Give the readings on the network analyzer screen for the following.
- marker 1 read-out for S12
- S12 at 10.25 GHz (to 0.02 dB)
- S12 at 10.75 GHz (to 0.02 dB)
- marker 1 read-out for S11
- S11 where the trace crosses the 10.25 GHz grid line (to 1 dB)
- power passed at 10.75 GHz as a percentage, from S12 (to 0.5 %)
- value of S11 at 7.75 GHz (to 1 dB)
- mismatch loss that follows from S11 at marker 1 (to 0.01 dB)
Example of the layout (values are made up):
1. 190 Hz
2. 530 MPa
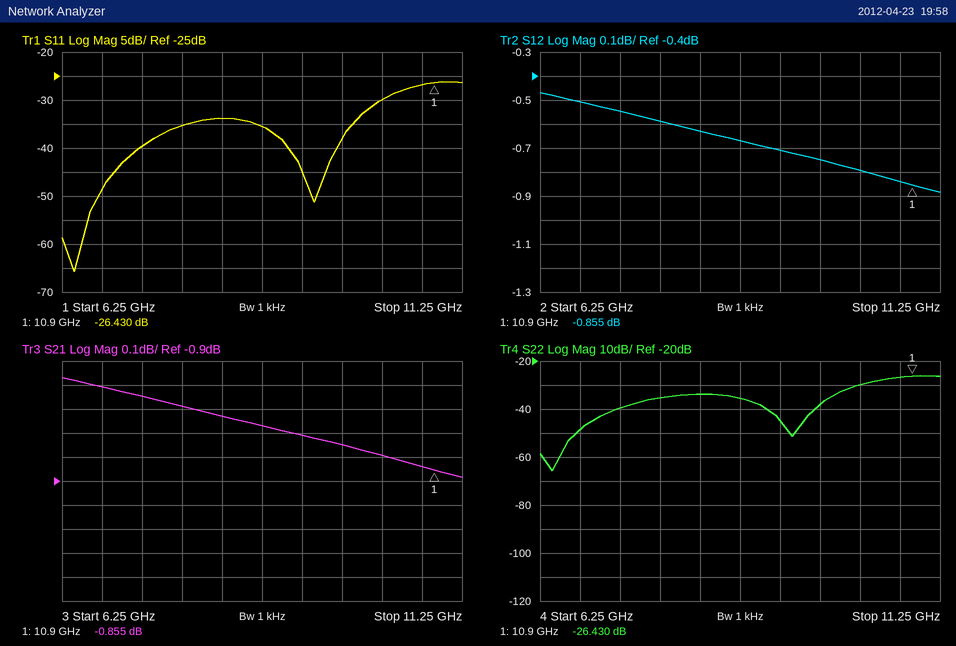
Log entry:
1. -0.855 dB
2. -0.80 dB
3. -0.84 dB
4. -26.430 dB
5. -30 dB
6. 82.5 %
7. -35 dB
8. 0.01 dB
